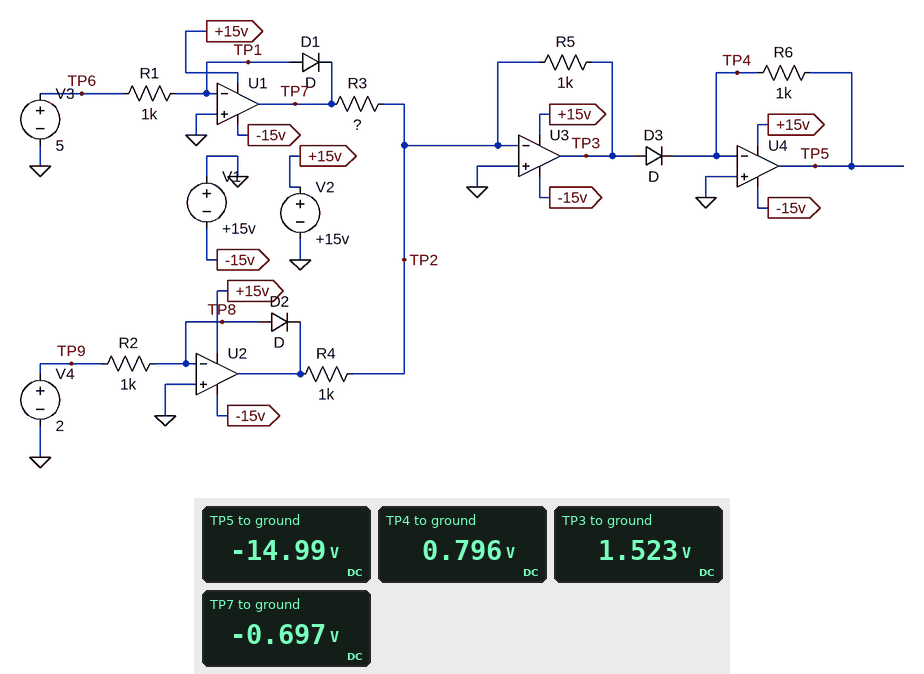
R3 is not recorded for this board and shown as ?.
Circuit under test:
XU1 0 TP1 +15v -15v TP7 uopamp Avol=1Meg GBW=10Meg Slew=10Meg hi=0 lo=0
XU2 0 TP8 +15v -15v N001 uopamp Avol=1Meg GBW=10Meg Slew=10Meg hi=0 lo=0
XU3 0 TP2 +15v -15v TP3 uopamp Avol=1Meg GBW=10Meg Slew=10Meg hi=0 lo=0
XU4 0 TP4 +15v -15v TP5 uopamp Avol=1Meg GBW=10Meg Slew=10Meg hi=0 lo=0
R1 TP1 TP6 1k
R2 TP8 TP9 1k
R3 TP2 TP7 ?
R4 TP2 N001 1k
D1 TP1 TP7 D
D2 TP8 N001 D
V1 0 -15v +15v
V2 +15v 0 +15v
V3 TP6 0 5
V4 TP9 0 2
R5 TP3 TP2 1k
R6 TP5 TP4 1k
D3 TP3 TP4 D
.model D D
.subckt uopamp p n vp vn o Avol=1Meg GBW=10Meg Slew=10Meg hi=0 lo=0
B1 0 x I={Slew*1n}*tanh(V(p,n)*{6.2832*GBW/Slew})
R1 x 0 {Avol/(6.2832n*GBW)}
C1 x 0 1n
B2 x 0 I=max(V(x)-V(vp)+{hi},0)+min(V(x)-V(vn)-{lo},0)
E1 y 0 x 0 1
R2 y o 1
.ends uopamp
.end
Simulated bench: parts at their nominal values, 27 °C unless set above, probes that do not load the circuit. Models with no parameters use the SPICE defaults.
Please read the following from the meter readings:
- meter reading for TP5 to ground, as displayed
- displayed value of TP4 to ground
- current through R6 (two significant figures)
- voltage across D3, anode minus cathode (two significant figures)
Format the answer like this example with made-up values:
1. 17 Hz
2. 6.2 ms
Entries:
1. -14.99 V
2. 0.796 V
3. 16 mA
4. 730 mV
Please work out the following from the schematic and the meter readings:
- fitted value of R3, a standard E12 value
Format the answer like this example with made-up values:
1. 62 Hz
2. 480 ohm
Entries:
1. 820 Ω
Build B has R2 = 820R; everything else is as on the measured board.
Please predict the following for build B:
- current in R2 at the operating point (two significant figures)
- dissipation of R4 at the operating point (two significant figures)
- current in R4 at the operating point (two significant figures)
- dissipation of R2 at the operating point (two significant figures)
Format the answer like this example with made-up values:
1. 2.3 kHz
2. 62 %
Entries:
1. 2.4 mA
2. 460 µW
3. 680 µA
4. 4.9 mW
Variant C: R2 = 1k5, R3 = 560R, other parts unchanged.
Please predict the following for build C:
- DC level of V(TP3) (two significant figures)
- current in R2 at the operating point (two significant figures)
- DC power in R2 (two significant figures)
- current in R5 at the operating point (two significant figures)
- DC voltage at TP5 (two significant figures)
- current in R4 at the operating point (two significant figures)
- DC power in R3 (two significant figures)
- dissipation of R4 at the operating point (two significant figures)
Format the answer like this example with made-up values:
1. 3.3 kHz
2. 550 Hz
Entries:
1. 1.9 V
2. 1.3 mA
3. 2.7 mW
4. 1.9 mA
5. -15 V
6. 660 µA
7. 870 µW
8. 440 µW
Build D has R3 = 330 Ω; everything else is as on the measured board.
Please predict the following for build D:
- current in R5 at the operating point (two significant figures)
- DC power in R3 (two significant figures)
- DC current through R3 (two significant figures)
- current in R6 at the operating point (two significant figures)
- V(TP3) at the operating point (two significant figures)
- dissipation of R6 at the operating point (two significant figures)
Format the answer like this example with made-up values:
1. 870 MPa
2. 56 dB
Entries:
1. 2.8 mA
2. 1.5 mW
3. 2.1 mA
4. 17 mA
5. 2.8 V
6. 290 mW
